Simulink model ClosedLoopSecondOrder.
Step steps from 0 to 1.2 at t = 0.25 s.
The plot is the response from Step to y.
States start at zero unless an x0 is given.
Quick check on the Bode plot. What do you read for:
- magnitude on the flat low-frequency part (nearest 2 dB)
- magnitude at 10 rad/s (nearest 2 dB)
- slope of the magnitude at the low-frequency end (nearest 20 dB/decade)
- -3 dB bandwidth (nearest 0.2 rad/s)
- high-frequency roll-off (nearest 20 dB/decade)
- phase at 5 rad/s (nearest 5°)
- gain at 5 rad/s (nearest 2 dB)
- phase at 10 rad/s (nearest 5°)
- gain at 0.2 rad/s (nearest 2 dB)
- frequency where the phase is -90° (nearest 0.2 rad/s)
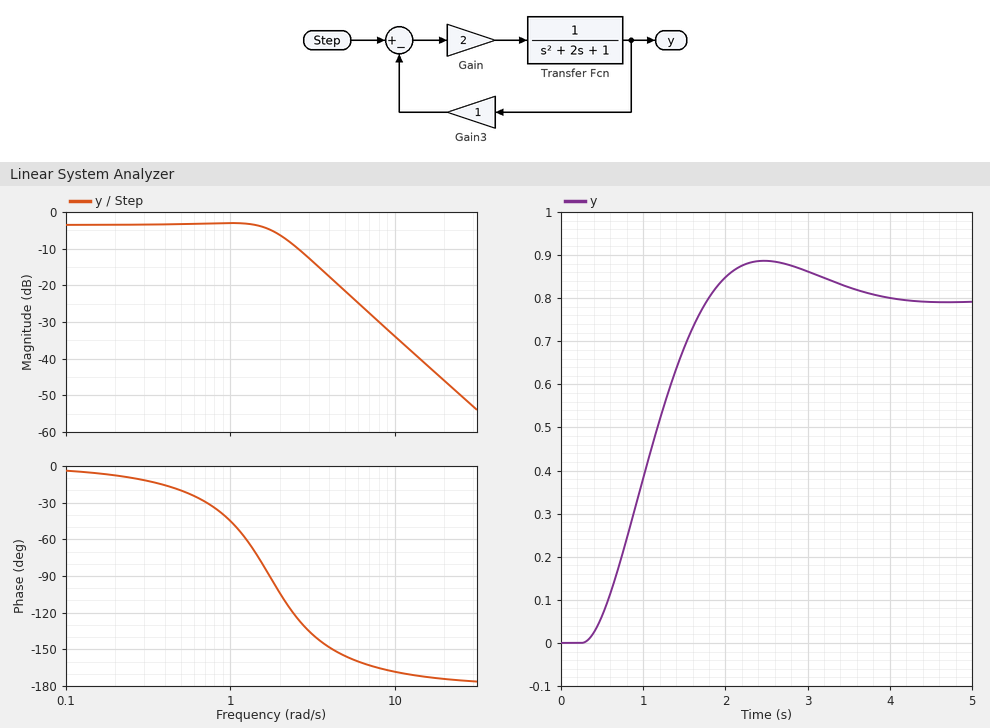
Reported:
-4 dB
-34 dB
0 dB/decade
2.0 rad/s
-40 dB/decade
-155°
-22 dB
-170°
-4 dB
1.8 rad/s
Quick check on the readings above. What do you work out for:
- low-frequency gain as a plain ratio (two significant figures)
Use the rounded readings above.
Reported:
0.63
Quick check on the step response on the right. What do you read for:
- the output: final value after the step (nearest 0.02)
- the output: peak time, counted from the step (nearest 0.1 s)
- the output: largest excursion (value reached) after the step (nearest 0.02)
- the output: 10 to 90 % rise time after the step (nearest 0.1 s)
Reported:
0.80
2.2 s
0.88
1.0 s
